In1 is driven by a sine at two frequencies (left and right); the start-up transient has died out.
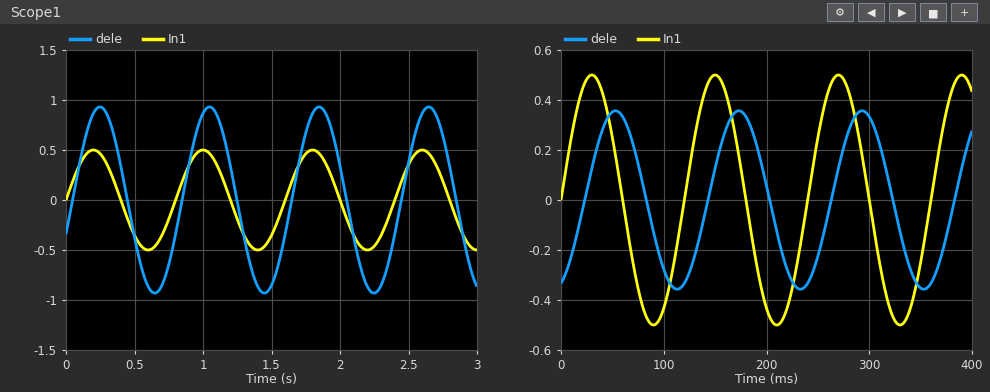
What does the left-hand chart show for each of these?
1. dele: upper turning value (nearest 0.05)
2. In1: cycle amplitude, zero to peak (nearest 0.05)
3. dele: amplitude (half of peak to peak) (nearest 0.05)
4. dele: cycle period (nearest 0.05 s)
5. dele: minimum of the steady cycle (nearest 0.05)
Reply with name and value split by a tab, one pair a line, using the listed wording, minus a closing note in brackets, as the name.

dele: upper turning value	0.95
In1: cycle amplitude, zero to peak	0.50
dele: amplitude (half of peak to peak)	0.95
dele: cycle period	0.80 s
dele: minimum of the steady cycle	-0.95
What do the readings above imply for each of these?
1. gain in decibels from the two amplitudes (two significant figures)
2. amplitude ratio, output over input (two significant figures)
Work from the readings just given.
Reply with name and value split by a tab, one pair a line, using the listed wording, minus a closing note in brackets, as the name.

gain in decibels from the two amplitudes	5.6 dB
amplitude ratio, output over input	1.9
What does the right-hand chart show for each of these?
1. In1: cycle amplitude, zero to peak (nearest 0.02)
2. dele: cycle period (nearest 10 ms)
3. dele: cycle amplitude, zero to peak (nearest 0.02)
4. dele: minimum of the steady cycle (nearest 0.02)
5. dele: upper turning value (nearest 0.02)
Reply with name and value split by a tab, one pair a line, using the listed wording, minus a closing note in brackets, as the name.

In1: cycle amplitude, zero to peak	0.50
dele: cycle period	120 ms
dele: cycle amplitude, zero to peak	0.36
dele: minimum of the steady cycle	-0.36
dele: upper turning value	0.36
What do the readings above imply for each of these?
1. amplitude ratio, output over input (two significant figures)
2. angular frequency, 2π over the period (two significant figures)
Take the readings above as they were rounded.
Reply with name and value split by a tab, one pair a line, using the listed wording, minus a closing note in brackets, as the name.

amplitude ratio, output over input	0.72
angular frequency, 2π over the period	0.052 rad/ms
